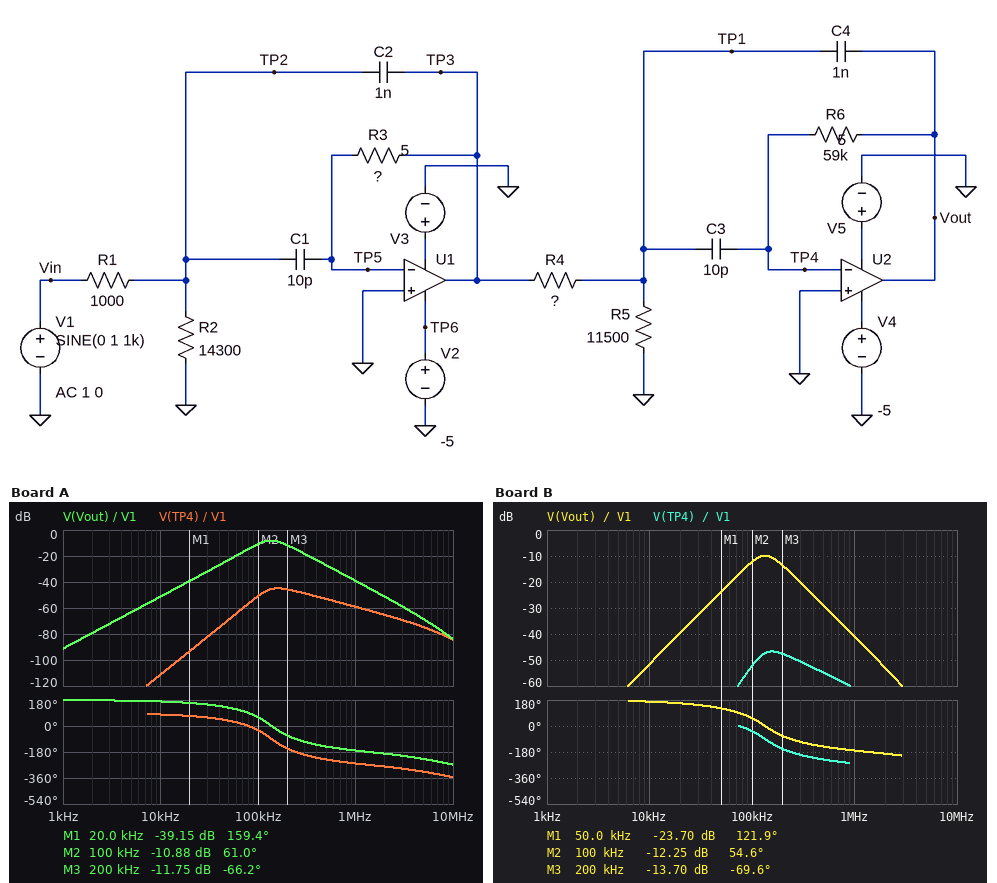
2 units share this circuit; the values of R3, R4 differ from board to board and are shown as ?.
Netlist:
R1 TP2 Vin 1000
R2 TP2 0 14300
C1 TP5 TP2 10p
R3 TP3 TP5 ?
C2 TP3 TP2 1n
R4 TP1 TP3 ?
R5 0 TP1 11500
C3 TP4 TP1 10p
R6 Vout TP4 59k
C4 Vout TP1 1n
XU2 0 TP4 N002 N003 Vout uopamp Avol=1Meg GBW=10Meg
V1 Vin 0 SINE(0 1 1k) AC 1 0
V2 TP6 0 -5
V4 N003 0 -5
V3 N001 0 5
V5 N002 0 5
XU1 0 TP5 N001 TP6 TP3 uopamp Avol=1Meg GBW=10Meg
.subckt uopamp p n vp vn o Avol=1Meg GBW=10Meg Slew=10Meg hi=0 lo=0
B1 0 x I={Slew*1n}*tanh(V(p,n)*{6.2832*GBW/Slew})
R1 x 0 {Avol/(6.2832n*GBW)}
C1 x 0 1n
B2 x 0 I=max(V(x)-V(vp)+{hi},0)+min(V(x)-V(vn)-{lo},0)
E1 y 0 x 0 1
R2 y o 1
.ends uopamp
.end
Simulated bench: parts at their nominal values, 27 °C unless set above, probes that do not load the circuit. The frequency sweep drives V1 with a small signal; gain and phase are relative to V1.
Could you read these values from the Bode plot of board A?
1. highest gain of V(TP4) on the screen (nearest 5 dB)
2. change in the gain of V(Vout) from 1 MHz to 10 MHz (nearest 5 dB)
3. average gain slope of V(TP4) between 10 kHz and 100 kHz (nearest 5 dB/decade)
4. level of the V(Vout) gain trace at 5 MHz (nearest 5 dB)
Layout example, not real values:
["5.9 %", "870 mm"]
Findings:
["-45 dB", "-45 dB", "60 dB/decade", "-70 dB"]
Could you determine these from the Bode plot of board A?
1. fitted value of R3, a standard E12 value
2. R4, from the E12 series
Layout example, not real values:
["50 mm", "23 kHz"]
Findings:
["150 kΩ", "2.2 kΩ"]
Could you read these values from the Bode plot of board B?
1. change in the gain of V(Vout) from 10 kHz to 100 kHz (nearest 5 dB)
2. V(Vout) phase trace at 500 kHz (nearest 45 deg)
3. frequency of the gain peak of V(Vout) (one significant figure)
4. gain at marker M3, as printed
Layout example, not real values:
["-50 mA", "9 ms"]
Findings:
["40 dB", "-135 deg", "100 kHz", "-13.70 dB"]
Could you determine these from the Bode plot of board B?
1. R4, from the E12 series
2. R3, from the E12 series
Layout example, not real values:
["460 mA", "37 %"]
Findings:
["2.7 kΩ", "150 kΩ"]
